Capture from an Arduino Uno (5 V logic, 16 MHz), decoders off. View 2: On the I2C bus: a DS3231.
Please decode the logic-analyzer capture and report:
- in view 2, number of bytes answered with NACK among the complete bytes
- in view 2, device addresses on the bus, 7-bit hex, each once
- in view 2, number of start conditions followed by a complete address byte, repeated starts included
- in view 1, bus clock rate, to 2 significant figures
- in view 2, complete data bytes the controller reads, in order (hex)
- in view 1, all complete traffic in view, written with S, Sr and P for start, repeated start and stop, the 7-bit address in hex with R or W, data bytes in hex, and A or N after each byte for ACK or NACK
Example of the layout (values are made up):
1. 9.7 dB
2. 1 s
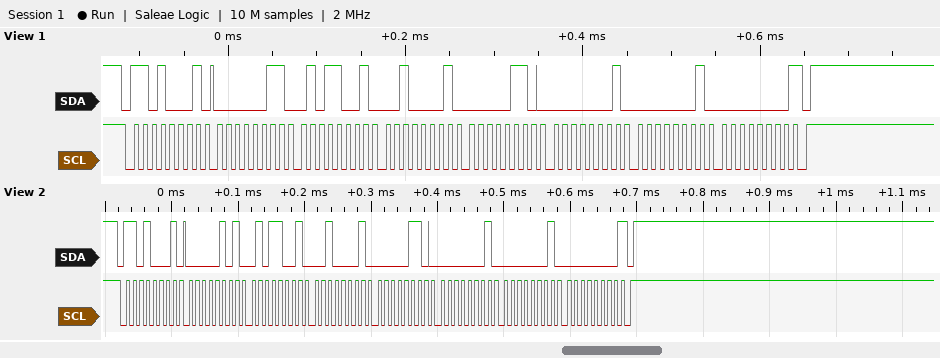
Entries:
1. 1
2. 0x68
3. 1
4. 100 kHz
5. 05 59 21 06 01 01 00
6. S 68R A 03 A 59 A 21 A 06 A 01 A 01 A 00 N P
